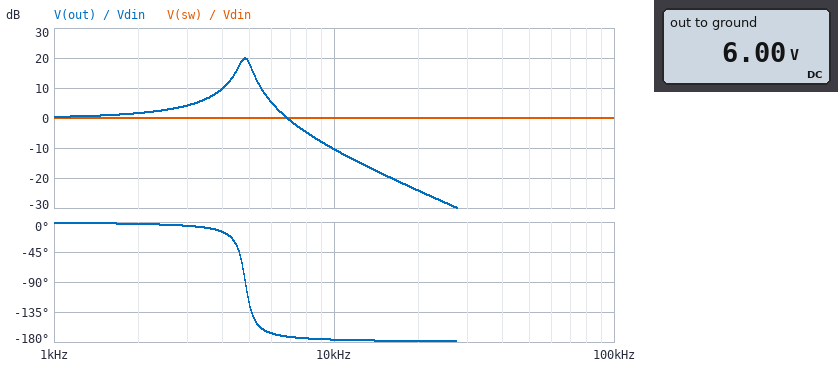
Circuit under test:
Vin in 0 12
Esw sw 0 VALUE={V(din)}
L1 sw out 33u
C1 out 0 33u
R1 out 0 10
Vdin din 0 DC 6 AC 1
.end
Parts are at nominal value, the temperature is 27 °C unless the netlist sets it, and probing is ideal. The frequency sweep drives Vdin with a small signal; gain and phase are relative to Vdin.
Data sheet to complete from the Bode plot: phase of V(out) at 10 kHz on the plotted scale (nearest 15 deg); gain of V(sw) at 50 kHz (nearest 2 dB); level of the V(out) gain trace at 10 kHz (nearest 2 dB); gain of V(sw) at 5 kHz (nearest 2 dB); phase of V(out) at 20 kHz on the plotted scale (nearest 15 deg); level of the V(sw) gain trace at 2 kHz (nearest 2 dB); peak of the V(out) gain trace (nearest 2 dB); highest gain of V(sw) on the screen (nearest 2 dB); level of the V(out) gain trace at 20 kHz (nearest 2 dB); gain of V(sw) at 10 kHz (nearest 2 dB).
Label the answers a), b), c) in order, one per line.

a) -180 deg
b) 0 dB
c) -10 dB
d) 0 dB
e) -180 deg
f) 0 dB
g) 20 dB
h) 0 dB
i) -24 dB
j) 0 dB
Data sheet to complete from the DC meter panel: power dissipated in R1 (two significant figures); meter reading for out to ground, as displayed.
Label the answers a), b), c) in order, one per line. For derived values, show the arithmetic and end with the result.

a) (6 V)^2 / 10 Ω = 3.6 W
b) 6.00 V
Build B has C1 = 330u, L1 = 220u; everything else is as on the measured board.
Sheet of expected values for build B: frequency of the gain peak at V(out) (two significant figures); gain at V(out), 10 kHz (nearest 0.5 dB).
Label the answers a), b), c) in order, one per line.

a) 590 Hz
b) -49.0 dB
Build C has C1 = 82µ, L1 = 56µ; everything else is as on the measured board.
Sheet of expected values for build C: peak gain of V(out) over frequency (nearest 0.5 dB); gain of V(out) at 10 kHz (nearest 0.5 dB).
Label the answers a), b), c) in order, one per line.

a) 21.5 dB
b) -24.5 dB
